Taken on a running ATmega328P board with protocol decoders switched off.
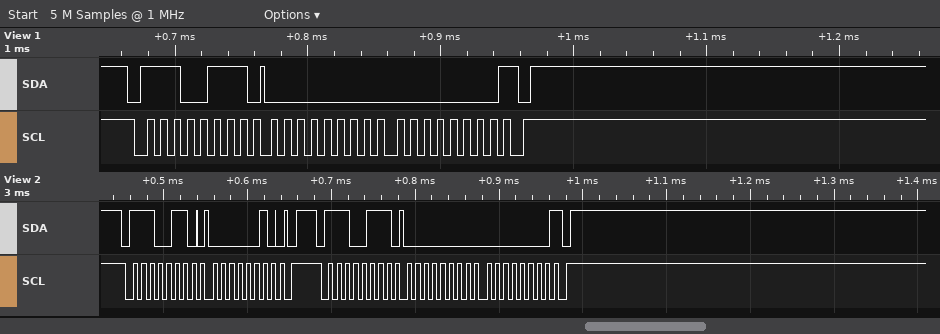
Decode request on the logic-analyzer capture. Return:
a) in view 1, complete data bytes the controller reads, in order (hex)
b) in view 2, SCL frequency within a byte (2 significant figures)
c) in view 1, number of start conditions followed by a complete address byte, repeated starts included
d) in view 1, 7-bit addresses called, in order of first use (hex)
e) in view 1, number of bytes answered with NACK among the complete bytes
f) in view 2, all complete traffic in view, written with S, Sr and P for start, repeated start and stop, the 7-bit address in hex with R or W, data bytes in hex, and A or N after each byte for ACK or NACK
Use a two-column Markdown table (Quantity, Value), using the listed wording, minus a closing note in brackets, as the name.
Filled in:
| Quantity | Value |
|---|---|
| in view 1, complete data bytes the controller reads, in order | 00 00 |
| in view 2, SCL frequency within a byte | 100 kHz |
| in view 1, number of start conditions followed by a complete address byte, repeated starts included | 1 |
| in view 1, 7-bit addresses called, in order of first use | 0x73 |
| in view 1, number of bytes answered with NACK among the complete bytes | 1 |
| in view 2, all complete traffic in view, written with S, Sr and P for start, repeated start and stop, the 7-bit address in hex with R or W, data bytes in hex, and A or N after each byte for ACK or NACK | S 73W A 02 A P S 73R A 00 A 00 N P |
